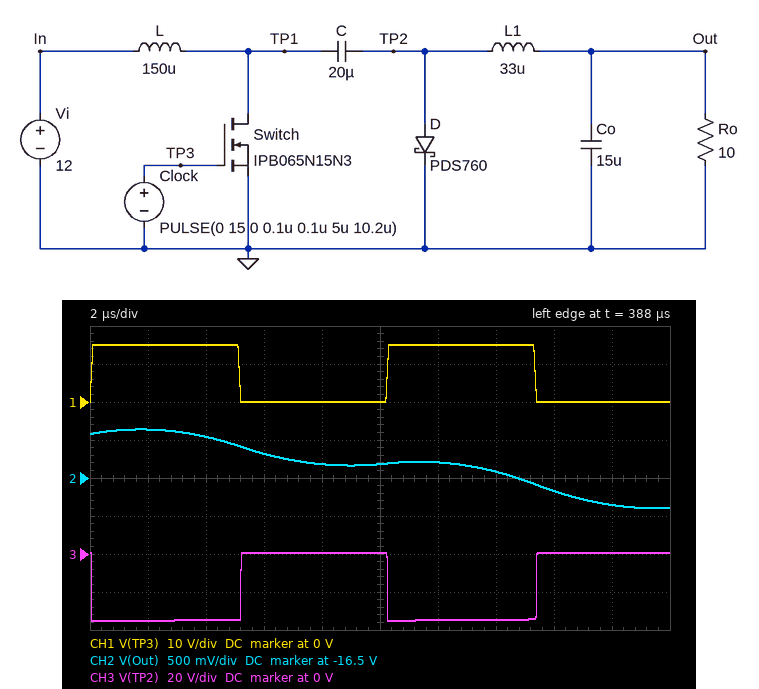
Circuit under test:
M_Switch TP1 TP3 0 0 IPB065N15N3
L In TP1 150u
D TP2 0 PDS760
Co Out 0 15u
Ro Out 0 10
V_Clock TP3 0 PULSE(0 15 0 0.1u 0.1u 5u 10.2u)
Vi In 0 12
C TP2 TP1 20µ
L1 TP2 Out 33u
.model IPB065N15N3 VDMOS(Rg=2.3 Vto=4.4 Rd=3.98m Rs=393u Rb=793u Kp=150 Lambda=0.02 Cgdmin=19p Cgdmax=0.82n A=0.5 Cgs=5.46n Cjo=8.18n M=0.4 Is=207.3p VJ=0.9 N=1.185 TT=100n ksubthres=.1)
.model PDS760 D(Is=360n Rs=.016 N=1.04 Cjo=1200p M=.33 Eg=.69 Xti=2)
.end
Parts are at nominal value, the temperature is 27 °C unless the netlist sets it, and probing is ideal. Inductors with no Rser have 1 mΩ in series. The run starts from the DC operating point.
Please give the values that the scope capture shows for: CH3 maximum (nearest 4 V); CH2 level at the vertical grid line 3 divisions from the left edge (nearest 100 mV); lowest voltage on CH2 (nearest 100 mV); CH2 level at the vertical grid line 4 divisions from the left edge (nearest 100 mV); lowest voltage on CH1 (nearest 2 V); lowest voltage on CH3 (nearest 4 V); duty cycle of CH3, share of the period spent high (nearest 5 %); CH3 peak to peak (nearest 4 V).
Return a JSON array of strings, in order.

["0 V", "-16.2 V", "-16.9 V", "-16.3 V", "0 V", "-36 V", "50 %", "36 V"]
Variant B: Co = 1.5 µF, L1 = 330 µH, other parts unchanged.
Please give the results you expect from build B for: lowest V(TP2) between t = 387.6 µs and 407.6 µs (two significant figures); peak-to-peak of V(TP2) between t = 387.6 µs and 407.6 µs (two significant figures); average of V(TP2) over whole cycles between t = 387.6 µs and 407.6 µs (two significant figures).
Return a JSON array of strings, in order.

["-33 V", "33 V", "-16 V"]
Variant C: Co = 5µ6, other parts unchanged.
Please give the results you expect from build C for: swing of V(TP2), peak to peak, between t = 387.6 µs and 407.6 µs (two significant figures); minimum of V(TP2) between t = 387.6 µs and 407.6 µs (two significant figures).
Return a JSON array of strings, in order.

["34 V", "-34 V"]
